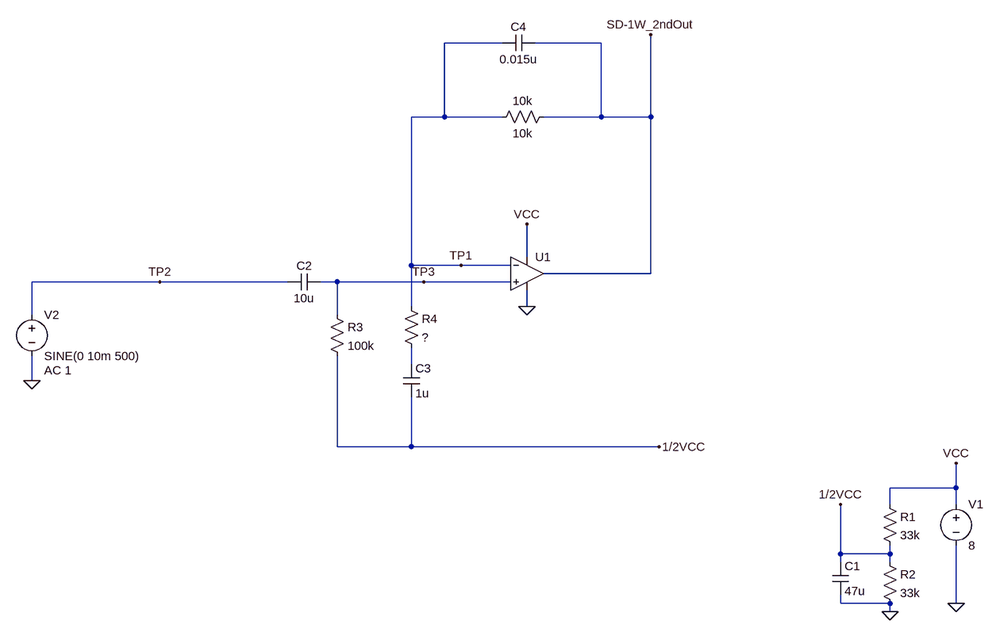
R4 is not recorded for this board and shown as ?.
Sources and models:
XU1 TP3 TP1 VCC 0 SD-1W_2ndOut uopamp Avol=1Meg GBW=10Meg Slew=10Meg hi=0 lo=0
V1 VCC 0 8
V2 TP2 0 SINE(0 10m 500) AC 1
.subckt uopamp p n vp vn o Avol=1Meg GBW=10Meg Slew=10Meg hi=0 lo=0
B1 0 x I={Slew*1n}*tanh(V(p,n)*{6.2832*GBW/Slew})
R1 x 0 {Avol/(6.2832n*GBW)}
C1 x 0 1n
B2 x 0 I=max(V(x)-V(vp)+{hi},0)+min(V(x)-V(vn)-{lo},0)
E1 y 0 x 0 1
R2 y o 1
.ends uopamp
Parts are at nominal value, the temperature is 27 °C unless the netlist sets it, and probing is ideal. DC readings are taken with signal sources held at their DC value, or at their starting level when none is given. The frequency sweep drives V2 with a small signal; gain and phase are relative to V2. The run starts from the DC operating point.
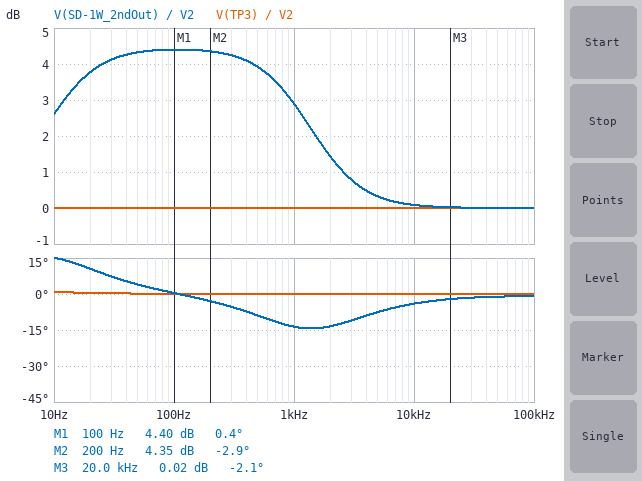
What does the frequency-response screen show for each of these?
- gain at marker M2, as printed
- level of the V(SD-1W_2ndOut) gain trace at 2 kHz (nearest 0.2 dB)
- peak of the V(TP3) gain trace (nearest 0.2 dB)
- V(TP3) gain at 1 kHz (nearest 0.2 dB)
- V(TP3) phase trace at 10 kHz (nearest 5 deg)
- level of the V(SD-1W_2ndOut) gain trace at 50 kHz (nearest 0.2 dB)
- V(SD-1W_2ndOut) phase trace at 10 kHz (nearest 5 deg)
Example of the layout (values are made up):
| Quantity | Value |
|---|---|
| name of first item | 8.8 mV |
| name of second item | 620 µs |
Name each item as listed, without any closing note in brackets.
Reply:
| Quantity | Value |
|---|---|
| gain at marker M2, as printed | 4.35 dB |
| level of the V(SD-1W_2ndOut) gain trace at 2 kHz | 1.4 dB |
| peak of the V(TP3) gain trace | 0 dB |
| V(TP3) gain at 1 kHz | 0 dB |
| V(TP3) phase trace at 10 kHz | 0 deg |
| level of the V(SD-1W_2ndOut) gain trace at 50 kHz | 0 dB |
| V(SD-1W_2ndOut) phase trace at 10 kHz | -5 deg |
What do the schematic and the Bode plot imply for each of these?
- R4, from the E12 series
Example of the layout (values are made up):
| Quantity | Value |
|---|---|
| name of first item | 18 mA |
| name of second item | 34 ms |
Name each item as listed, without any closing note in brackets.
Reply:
| Quantity | Value |
|---|---|
| R4, from the E12 series | 15 kΩ |
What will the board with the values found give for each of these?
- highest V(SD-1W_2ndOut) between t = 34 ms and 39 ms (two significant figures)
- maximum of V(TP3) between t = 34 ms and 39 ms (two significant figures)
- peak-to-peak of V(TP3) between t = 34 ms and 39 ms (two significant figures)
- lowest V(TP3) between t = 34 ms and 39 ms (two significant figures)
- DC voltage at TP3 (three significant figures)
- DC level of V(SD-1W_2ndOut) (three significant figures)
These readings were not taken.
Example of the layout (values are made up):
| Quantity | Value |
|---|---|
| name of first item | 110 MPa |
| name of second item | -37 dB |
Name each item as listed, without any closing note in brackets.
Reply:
| Quantity | Value |
|---|---|
| highest V(SD-1W_2ndOut) between t = 34 ms and 39 ms | 4.0 V |
| maximum of V(TP3) between t = 34 ms and 39 ms | 4.0 V |
| peak-to-peak of V(TP3) between t = 34 ms and 39 ms | 20 mV |
| lowest V(TP3) between t = 34 ms and 39 ms | 4.0 V |
| DC voltage at TP3 | 4.00 V |
| DC level of V(SD-1W_2ndOut) | 4.00 V |
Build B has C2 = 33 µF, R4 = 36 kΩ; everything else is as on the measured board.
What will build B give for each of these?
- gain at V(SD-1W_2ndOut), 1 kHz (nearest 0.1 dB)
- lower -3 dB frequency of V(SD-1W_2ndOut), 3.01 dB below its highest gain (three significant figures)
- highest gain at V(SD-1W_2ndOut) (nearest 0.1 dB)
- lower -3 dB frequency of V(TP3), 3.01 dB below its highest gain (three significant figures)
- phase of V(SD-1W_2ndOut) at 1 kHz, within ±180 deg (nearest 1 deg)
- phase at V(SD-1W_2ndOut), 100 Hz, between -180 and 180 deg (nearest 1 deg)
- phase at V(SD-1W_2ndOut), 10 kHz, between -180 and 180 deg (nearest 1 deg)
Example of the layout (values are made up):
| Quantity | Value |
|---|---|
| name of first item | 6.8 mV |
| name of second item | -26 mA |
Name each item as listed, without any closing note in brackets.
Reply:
| Quantity | Value |
|---|---|
| gain at V(SD-1W_2ndOut), 1 kHz | 1.3 dB |
| lower -3 dB frequency of V(SD-1W_2ndOut), 3.01 dB below its highest gain | 98.5 mHz |
| highest gain at V(SD-1W_2ndOut) | 2.1 dB |
| lower -3 dB frequency of V(TP3), 3.01 dB below its highest gain | 42.6 mHz |
| phase of V(SD-1W_2ndOut) at 1 kHz, within ±180 deg | -7 deg |
| phase at V(SD-1W_2ndOut), 100 Hz, between -180 and 180 deg | -1 deg |
| phase at V(SD-1W_2ndOut), 10 kHz, between -180 and 180 deg | -2 deg |
